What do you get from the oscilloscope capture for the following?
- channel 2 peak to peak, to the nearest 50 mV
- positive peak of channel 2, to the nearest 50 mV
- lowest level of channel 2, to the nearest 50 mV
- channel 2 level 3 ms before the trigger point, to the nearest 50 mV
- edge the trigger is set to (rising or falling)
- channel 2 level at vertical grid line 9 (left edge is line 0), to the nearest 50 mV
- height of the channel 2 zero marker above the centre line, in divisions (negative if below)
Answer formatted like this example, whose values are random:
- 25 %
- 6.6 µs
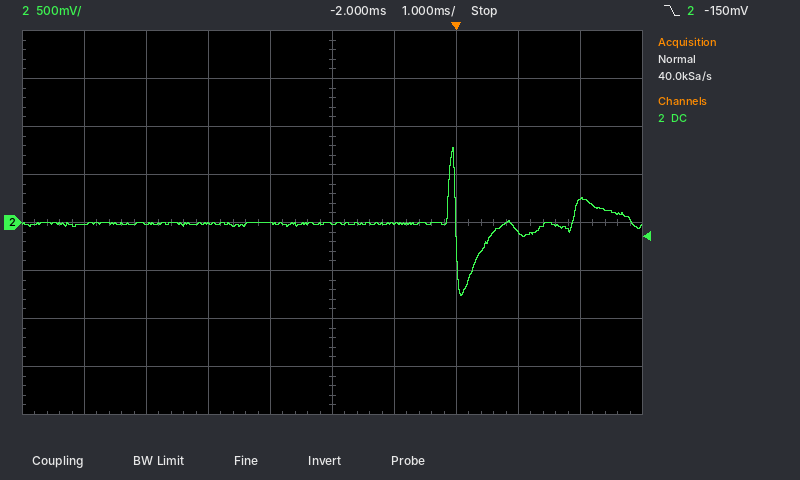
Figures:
- 1.55 V
- 800 mV
- -750 mV
- 0 mV
- falling
- 250 mV
- 0.0 div
